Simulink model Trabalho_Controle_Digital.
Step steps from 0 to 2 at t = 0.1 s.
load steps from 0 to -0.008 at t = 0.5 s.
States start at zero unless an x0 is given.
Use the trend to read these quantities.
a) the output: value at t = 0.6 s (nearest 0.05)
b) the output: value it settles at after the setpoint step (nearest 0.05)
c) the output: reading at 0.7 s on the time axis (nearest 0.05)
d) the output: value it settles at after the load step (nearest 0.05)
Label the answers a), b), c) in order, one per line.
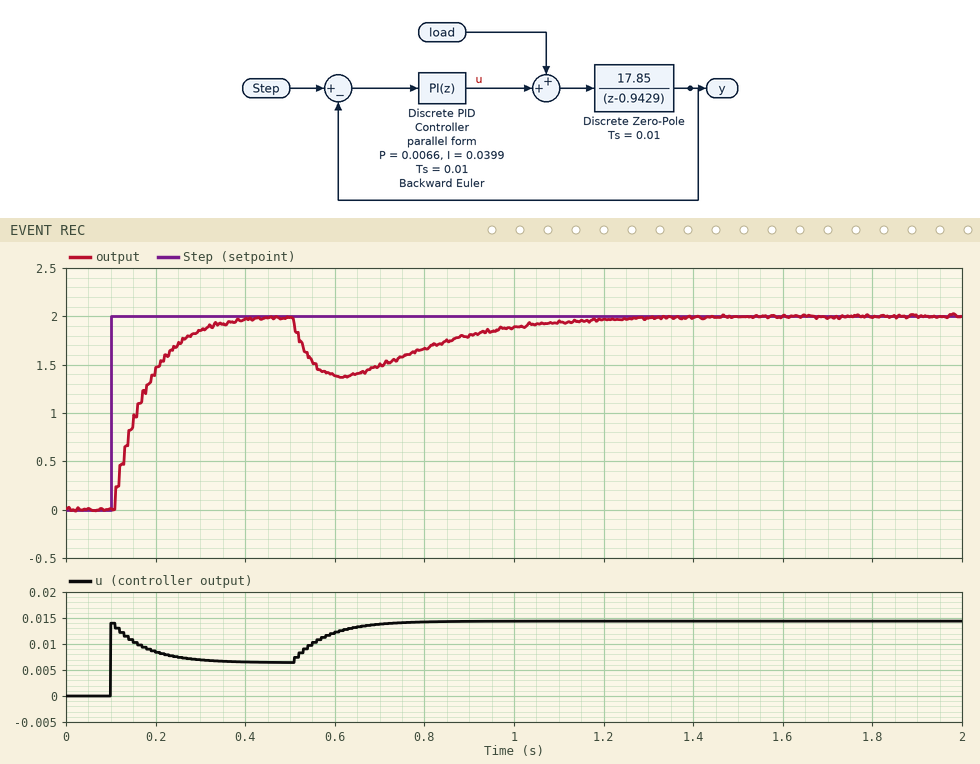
a) 1.40
b) 2.00
c) 1.50
d) 2.00
